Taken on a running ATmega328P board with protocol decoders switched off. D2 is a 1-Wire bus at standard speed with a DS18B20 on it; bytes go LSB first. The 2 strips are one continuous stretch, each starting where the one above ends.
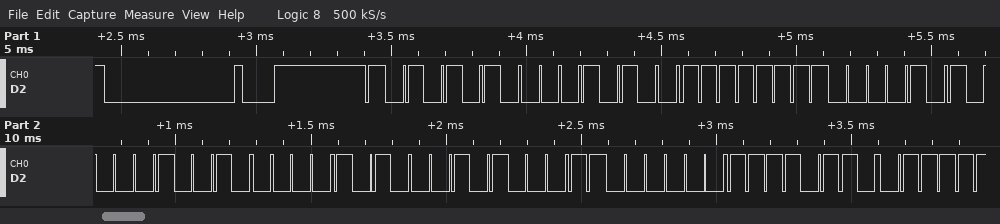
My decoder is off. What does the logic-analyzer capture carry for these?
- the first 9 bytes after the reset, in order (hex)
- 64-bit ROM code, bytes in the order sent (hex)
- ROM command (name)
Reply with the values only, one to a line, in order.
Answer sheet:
55 28 FF 50 48 50 14 03 6F
28 FF 50 48 50 14 03 6F
Match ROM
